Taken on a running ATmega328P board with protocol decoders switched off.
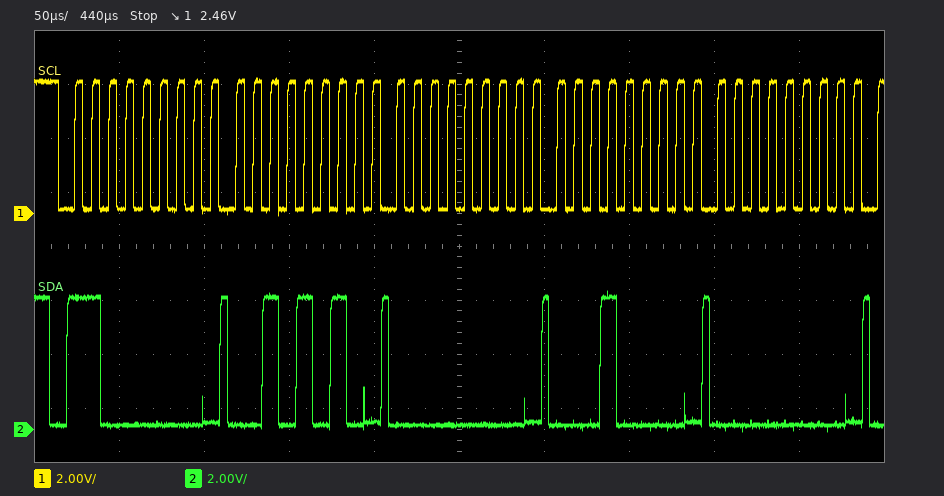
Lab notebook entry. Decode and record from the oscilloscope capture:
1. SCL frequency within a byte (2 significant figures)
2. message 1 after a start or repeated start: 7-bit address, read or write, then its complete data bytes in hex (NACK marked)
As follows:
100 kHz
0x60 write: 2A 00 10 00
